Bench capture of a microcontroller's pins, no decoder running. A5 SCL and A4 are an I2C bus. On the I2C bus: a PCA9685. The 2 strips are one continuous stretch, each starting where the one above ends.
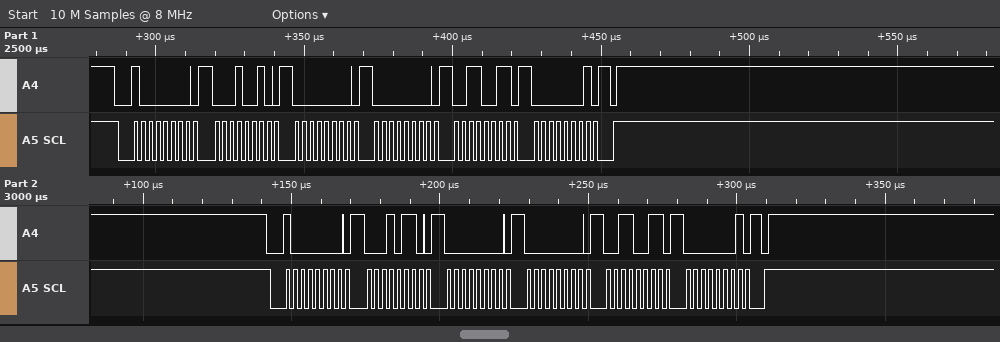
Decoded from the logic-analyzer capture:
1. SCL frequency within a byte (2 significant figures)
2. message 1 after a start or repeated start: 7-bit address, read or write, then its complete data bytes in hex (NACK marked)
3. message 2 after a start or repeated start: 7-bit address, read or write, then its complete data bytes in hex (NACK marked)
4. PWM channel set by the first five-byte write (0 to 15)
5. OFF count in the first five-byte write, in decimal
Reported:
400 kHz
0x40 write: 12 00 00 33 01
0x40 write: 16 00 00 33 01
3
307
